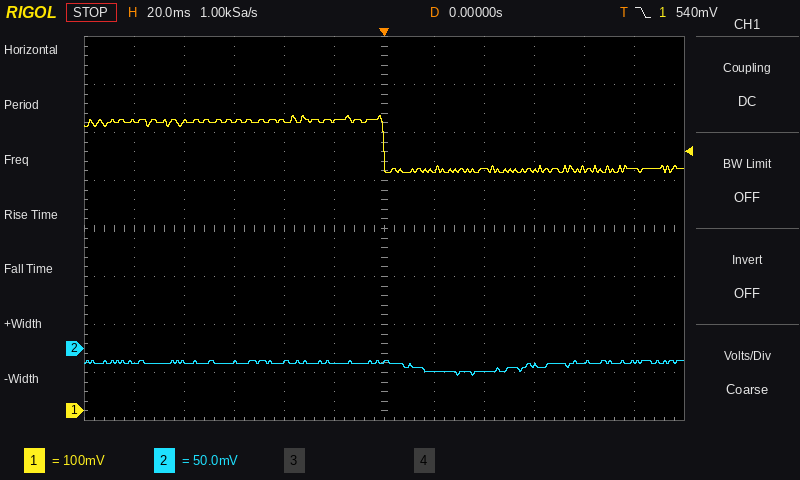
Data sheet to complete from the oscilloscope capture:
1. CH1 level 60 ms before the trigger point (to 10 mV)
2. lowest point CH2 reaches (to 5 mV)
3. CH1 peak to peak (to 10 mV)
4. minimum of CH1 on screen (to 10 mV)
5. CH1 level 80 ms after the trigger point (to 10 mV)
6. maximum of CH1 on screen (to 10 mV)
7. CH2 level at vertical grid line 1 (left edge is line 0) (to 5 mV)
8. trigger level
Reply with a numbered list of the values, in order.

1. 600 mV
2. -30 mV
3. 120 mV
4. 500 mV
5. 500 mV
6. 620 mV
7. -15 mV
8. 540 mV
